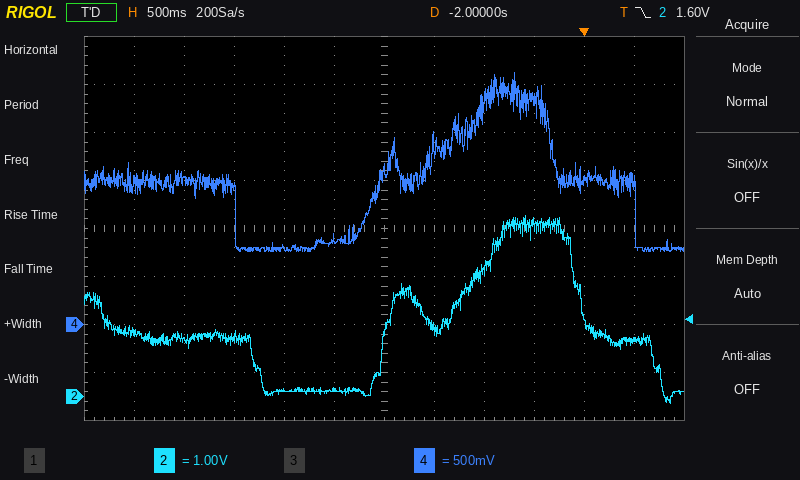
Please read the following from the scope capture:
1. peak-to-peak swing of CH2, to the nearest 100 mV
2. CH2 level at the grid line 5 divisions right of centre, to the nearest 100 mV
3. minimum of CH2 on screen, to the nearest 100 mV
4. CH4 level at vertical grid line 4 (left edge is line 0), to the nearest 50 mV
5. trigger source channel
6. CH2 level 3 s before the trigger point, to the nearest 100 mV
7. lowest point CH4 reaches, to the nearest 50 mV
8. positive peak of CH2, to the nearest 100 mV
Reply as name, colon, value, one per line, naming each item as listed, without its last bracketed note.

peak-to-peak swing of CH2, to the nearest 100 mV: 3.9 V
CH2 level at the grid line 5 divisions right of centre, to the nearest 100 mV: 1.2 V
minimum of CH2 on screen, to the nearest 100 mV: -100 mV
CH4 level at vertical grid line 4 (left edge is line 0), to the nearest 50 mV: 800 mV
trigger source channel: CH2
CH2 level 3 s before the trigger point, to the nearest 100 mV: 100 mV
lowest point CH4 reaches, to the nearest 50 mV: 750 mV
positive peak of CH2, to the nearest 100 mV: 3.8 V
